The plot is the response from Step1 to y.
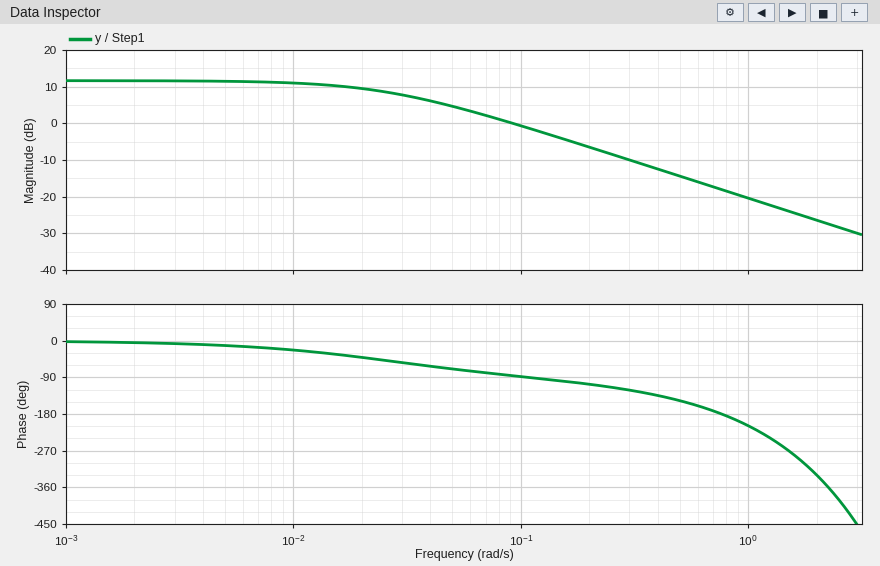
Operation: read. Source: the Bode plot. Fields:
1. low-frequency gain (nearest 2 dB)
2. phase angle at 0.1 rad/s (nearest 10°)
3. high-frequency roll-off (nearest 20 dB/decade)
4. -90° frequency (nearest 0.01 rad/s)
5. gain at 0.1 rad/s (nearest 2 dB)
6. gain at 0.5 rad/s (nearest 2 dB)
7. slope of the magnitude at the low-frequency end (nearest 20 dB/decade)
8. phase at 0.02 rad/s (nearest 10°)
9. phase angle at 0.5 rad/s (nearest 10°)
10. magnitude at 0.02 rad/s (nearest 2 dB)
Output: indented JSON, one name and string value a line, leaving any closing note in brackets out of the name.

{
  "low-frequency gain": "12 dB",
  "phase angle at 0.1 rad/s": "-90°",
  "high-frequency roll-off": "-20 dB/decade",
  "-90° frequency": "0.11 rad/s",
  "gain at 0.1 rad/s": "0 dB",
  "gain at 0.5 rad/s": "-14 dB",
  "slope of the magnitude at the low-frequency end": "0 dB/decade",
  "phase at 0.02 rad/s": "-40°",
  "phase angle at 0.5 rad/s": "-150°",
  "magnitude at 0.02 rad/s": "10 dB"
}
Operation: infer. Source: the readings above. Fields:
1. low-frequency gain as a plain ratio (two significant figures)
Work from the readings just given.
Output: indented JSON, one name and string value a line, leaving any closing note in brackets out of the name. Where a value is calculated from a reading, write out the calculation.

{
  "low-frequency gain as a plain ratio": "10^(12 / 20) = 4.0"
}
